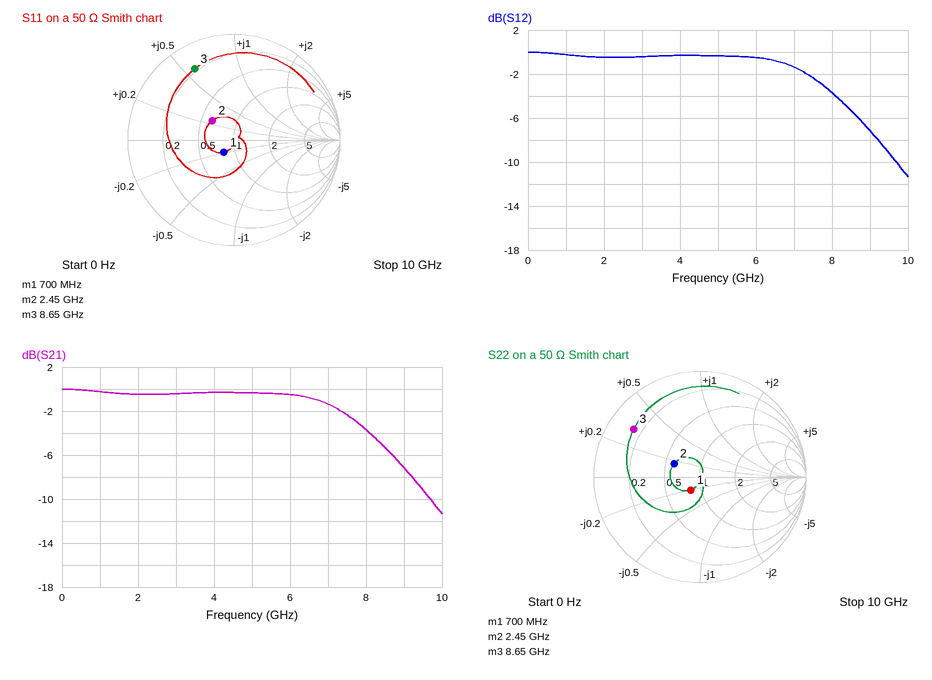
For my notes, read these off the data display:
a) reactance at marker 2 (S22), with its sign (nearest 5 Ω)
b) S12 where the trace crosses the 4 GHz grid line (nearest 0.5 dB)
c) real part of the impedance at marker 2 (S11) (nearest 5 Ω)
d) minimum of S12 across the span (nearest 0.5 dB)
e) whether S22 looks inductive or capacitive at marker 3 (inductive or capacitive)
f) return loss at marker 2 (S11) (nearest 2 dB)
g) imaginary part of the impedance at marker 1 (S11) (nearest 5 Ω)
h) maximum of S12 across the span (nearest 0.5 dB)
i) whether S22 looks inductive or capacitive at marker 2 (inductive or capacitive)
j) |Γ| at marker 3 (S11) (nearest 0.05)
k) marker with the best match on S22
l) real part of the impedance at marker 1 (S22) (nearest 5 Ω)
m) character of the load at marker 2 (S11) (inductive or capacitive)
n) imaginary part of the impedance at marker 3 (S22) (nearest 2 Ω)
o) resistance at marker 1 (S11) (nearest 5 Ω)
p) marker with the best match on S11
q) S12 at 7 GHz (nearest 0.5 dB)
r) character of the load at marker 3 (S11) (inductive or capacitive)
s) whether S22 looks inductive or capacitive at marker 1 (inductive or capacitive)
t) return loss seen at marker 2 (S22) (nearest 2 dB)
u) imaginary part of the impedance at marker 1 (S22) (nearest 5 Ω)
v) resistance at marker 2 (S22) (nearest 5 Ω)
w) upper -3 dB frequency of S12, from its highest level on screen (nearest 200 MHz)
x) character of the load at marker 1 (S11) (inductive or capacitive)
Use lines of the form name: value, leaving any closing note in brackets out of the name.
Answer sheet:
reactance at marker 2 (S22), with its sign: +10 Ω
S12 where the trace crosses the 4 GHz grid line: -0.5 dB
real part of the impedance at marker 2 (S11): 30 Ω
minimum of S12 across the span: -11.5 dB
whether S22 looks inductive or capacitive at marker 3: inductive
return loss at marker 2 (S11): 12 dB
imaginary part of the impedance at marker 1 (S11): -10 Ω
maximum of S12 across the span: 0.0 dB
whether S22 looks inductive or capacitive at marker 2: inductive
|Γ| at marker 3 (S11): 0.75
marker with the best match on S22: marker 1
real part of the impedance at marker 1 (S22): 40 Ω
character of the load at marker 2 (S11): inductive
imaginary part of the impedance at marker 3 (S22): +16 Ω
resistance at marker 1 (S11): 40 Ω
marker with the best match on S11: marker 1
S12 at 7 GHz: -1.5 dB
character of the load at marker 3 (S11): inductive
whether S22 looks inductive or capacitive at marker 1: capacitive
return loss seen at marker 2 (S22): 12 dB
imaginary part of the impedance at marker 1 (S22): -10 Ω
resistance at marker 2 (S22): 30 Ω
upper -3 dB frequency of S12, from its highest level on screen: 7.8 GHz
character of the load at marker 1 (S11): capacitive
